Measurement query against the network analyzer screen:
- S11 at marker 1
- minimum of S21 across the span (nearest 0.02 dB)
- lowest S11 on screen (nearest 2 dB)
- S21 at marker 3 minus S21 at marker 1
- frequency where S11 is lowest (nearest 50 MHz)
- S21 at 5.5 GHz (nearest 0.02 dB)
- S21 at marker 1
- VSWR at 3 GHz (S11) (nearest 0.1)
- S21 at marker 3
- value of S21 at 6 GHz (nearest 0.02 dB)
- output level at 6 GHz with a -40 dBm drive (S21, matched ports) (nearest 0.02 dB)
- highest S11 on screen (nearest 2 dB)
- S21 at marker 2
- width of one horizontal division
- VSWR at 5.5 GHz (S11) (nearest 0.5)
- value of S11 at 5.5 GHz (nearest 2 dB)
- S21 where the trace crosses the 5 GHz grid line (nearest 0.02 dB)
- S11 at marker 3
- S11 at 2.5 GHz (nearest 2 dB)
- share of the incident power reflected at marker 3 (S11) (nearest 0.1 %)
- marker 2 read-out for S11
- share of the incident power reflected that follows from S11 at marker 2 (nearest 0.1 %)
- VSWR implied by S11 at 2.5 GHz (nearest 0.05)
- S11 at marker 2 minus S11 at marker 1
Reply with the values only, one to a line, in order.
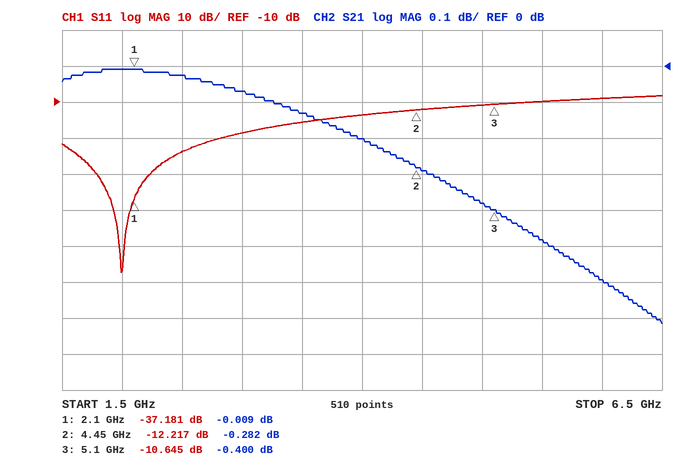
-37.181 dB
-0.72 dB
-58 dB
-0.391 dB
2.00 GHz
-0.48 dB
-0.009 dB
1.3
-0.400 dB
-0.60 dB
-40.60 dBm
-8 dB
-0.282 dB
500 MHz
2.0
-10 dB
-0.38 dB
-10.645 dB
-24 dB
8.6 %
-12.217 dB
6.0 %
1.15
24.964 dB
